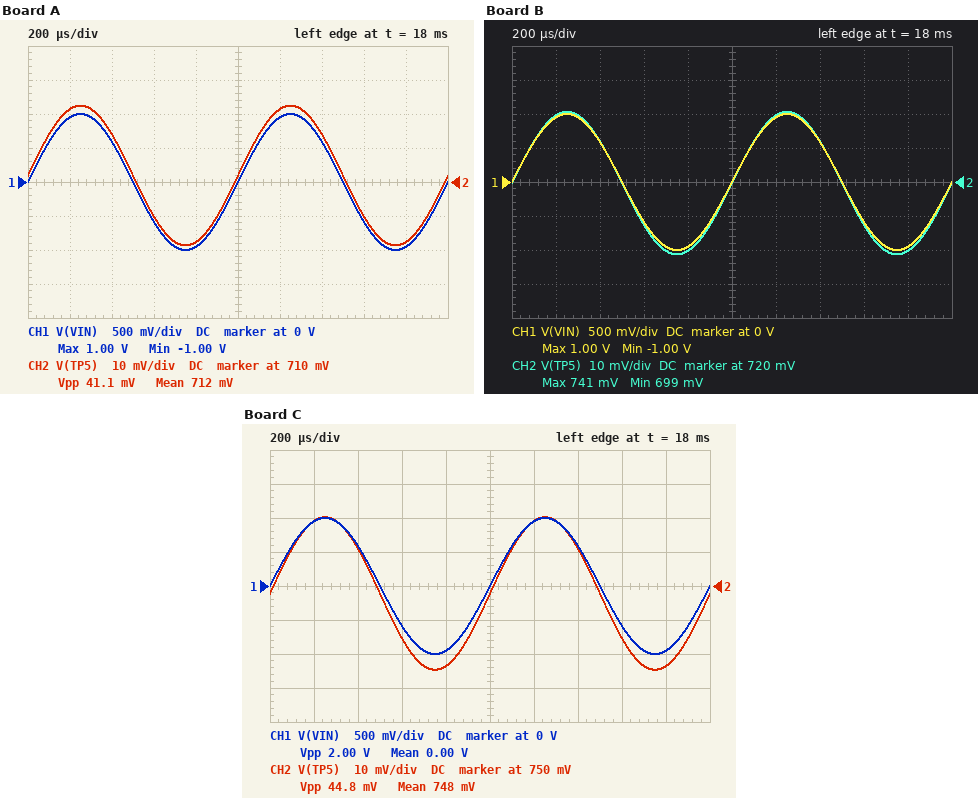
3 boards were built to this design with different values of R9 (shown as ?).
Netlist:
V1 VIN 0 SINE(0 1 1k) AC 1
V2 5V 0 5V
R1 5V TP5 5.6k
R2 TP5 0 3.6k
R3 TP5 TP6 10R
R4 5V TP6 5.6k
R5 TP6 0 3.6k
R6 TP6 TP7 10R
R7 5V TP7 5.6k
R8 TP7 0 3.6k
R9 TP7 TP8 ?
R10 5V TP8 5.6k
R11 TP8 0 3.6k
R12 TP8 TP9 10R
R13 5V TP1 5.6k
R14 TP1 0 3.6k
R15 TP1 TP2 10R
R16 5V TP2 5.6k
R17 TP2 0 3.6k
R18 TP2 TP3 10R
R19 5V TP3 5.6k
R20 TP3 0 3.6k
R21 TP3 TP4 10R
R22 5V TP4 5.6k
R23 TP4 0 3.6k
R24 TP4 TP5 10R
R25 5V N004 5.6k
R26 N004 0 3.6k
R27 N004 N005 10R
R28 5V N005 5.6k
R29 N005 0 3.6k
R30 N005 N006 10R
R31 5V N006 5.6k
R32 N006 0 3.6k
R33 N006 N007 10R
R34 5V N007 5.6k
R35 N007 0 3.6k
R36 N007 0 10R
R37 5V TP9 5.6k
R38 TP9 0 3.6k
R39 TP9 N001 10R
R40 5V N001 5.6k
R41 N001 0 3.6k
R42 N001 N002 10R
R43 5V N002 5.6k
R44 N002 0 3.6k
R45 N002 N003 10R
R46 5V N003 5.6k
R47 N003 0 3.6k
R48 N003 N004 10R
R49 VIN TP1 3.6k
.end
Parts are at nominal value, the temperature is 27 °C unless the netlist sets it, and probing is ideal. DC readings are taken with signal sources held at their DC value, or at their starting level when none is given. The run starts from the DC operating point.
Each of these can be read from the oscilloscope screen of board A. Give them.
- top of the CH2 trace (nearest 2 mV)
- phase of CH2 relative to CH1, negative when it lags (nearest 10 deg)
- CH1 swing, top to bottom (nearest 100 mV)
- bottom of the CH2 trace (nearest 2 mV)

732 mV
0 deg
2.0 V
692 mV
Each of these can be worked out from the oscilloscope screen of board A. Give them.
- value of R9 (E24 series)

4.7 Ω
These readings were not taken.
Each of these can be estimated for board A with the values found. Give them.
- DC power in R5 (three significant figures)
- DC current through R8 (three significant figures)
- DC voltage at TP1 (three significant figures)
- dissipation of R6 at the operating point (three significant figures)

131 µW
182 µA
758 mV
98.8 µW
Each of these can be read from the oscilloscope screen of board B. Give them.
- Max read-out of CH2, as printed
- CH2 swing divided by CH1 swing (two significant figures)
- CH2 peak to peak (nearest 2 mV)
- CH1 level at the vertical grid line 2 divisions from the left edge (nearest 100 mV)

741 mV
0.021
42 mV
600 mV
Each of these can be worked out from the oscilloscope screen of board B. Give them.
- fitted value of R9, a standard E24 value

7.5 Ω
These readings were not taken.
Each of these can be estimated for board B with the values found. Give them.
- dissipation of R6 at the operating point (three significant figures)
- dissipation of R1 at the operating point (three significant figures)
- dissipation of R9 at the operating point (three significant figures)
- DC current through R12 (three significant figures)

97.4 µW
3.27 mW
103 µW
4.31 mA
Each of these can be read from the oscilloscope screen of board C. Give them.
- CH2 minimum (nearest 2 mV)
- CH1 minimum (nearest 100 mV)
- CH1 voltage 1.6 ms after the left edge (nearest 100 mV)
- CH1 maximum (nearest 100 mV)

726 mV
-1.0 V
-600 mV
1.0 V
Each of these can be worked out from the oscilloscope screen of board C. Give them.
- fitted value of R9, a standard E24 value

18 Ω
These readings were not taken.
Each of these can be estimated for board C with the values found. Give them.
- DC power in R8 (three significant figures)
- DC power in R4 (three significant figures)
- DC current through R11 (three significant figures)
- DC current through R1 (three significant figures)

133 µW
3.27 mW
174 µA
759 µA
